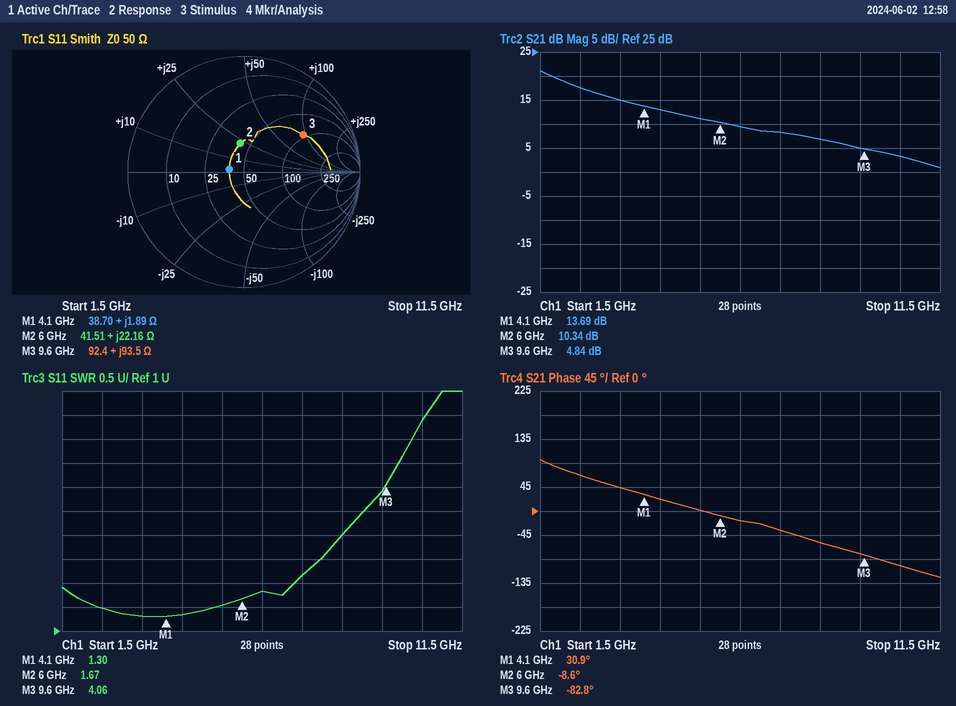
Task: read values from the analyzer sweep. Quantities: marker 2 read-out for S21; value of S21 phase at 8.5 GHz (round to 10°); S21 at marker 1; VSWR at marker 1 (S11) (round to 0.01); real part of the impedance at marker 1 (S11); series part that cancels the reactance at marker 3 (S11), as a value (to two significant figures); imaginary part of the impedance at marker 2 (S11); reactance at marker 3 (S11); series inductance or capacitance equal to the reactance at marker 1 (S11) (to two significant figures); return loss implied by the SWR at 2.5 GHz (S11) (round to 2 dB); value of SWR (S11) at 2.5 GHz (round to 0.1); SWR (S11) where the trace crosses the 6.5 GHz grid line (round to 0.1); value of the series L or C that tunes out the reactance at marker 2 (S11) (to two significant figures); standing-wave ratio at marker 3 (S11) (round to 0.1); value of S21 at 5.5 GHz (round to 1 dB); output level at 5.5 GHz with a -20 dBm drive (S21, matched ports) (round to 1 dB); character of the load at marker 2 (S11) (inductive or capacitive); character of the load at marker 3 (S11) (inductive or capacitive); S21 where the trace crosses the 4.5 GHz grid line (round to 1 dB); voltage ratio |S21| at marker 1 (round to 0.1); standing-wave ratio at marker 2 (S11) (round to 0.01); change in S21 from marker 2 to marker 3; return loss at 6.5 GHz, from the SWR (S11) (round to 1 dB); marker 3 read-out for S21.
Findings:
10.34 dB
-60°
13.69 dB
1.30
38.70 Ω
180 fF
+22.16 Ω
+93.5 Ω
73 pH
14 dB
1.5
1.8
1.2 pF
4.0
11 dB
-9 dBm
inductive
inductive
13 dB
4.8
1.67
-5.50 dB
11 dB
4.84 dB
